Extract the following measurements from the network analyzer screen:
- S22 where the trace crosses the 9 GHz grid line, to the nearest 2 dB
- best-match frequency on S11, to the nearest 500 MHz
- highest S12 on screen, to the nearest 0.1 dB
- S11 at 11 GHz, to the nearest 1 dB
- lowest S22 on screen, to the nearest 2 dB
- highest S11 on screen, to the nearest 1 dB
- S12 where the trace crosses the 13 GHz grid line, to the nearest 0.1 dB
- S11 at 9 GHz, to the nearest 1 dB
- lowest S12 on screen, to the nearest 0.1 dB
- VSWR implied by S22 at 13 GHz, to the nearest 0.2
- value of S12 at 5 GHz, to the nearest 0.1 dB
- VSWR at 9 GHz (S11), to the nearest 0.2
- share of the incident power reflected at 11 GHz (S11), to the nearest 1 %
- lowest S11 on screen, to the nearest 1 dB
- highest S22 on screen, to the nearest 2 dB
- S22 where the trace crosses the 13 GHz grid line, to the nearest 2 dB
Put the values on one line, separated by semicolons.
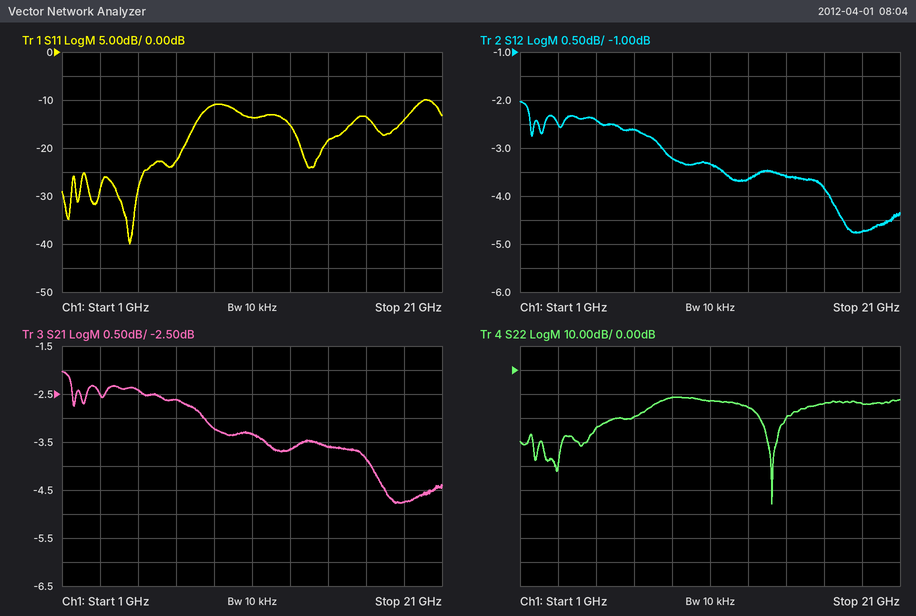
-12 dB; 4.5 GHz; -2.0 dB; -14 dB; -56 dB; -10 dB; -3.7 dB; -11 dB; -4.8 dB; 1.4; -2.4 dB; 1.8; 4 %; -40 dB; -12 dB; -16 dB
